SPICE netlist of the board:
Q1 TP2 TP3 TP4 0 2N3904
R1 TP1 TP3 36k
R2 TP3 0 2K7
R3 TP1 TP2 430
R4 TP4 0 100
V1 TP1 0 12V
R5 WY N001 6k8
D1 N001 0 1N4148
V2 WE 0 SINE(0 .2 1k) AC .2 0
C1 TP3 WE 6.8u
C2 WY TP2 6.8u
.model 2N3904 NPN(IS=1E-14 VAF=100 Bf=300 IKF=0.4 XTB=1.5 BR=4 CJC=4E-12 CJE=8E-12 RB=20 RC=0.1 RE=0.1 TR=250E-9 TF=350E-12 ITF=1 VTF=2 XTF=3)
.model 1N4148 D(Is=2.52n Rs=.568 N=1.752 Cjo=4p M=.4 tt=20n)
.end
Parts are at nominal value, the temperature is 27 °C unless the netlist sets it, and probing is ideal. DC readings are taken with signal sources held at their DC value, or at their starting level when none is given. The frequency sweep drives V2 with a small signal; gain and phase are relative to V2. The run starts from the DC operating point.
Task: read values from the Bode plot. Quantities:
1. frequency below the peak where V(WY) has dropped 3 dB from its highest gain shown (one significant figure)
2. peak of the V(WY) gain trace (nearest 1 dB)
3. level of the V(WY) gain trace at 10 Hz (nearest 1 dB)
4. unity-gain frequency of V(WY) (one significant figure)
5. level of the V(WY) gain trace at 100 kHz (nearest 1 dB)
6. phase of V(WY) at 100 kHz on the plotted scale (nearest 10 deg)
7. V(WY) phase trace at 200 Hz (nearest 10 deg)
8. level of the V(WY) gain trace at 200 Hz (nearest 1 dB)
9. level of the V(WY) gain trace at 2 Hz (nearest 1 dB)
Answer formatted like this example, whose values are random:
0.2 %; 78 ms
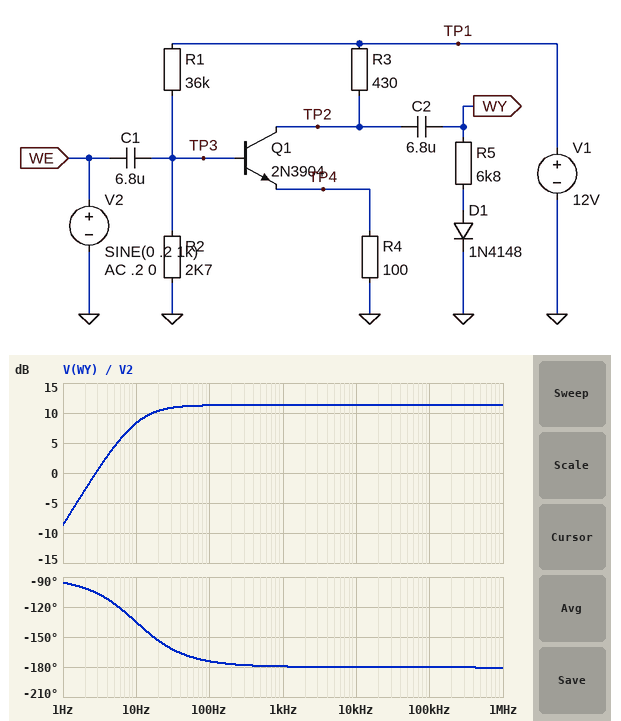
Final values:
10 Hz; 11 dB; 8 dB; 3 Hz; 11 dB; -180 deg; -180 deg; 11 dB; -3 dB
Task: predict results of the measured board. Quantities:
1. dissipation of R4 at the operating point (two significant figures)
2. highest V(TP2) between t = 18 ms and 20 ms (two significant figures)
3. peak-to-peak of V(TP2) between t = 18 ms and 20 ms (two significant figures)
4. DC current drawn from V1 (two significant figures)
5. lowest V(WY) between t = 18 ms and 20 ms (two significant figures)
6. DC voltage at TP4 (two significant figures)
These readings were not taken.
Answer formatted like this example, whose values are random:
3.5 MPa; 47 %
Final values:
260 µW; 12 V; 1.4 V; 1.9 mA; -780 mV; 160 mV
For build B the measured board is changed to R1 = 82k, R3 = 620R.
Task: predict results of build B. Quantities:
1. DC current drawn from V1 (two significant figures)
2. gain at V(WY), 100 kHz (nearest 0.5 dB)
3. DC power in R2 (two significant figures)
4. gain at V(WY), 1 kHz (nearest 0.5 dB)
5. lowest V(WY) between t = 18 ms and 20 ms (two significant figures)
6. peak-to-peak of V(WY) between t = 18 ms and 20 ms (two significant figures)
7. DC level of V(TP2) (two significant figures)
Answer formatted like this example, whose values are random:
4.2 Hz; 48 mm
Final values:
140 µA; -60.5 dB; 54 µW; -63.0 dB; -33 mV; 33 mV; 12 V
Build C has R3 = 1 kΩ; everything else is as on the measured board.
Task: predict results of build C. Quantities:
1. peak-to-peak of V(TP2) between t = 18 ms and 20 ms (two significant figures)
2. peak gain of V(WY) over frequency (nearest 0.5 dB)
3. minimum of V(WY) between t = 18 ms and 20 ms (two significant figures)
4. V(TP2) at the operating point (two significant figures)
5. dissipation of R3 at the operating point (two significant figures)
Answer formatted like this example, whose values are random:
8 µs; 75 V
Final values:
3.1 V; 18.5 dB; -1.9 V; 10 V; 2.5 mW
